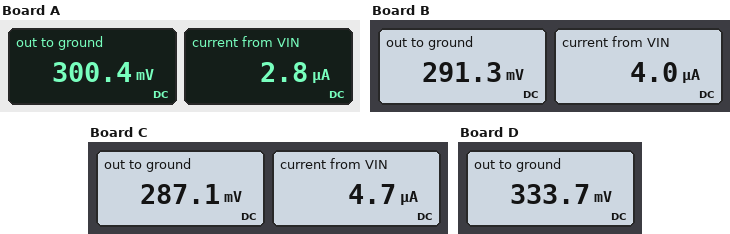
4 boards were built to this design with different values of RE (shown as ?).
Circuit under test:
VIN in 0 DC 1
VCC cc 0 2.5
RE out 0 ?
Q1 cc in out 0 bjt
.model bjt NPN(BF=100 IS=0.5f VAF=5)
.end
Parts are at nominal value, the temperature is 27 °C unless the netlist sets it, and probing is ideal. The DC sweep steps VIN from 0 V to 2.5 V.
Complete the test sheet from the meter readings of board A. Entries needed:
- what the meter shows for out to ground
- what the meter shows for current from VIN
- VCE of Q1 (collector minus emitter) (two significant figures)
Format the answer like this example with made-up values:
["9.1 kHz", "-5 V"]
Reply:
["300.4 mV", "2.8 µA", "2.2 V"]
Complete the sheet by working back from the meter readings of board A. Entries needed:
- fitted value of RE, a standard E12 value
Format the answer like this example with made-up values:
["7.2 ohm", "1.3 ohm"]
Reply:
["820 Ω"]
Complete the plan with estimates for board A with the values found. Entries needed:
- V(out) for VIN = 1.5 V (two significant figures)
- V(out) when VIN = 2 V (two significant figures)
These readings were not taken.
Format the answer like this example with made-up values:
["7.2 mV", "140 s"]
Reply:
["770 mV", "1.3 V"]
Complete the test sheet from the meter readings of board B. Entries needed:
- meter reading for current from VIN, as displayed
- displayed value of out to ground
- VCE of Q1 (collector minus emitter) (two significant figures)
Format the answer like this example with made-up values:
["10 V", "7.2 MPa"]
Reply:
["4.0 µA", "291.3 mV", "2.2 V"]
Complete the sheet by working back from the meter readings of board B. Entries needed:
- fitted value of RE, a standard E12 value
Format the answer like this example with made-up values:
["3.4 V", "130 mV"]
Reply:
["560 Ω"]
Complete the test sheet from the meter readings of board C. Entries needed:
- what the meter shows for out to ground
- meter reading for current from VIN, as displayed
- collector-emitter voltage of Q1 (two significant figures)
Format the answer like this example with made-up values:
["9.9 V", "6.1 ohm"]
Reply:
["287.1 mV", "4.7 µA", "2.2 V"]
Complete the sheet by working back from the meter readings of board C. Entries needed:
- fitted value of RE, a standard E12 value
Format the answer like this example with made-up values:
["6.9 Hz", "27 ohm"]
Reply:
["470 Ω"]
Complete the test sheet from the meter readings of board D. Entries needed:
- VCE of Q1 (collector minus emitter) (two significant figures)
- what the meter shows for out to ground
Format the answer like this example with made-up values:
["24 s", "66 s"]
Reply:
["2.2 V", "333.7 mV"]
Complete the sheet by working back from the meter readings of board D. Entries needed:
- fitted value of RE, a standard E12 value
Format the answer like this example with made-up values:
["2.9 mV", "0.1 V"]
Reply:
["3.3 kΩ"]
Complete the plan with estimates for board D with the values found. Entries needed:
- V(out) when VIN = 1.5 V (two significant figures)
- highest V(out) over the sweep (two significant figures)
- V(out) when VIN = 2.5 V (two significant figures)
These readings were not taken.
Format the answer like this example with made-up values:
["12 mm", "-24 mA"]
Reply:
["810 mV", "1.8 V", "1.8 V"]
